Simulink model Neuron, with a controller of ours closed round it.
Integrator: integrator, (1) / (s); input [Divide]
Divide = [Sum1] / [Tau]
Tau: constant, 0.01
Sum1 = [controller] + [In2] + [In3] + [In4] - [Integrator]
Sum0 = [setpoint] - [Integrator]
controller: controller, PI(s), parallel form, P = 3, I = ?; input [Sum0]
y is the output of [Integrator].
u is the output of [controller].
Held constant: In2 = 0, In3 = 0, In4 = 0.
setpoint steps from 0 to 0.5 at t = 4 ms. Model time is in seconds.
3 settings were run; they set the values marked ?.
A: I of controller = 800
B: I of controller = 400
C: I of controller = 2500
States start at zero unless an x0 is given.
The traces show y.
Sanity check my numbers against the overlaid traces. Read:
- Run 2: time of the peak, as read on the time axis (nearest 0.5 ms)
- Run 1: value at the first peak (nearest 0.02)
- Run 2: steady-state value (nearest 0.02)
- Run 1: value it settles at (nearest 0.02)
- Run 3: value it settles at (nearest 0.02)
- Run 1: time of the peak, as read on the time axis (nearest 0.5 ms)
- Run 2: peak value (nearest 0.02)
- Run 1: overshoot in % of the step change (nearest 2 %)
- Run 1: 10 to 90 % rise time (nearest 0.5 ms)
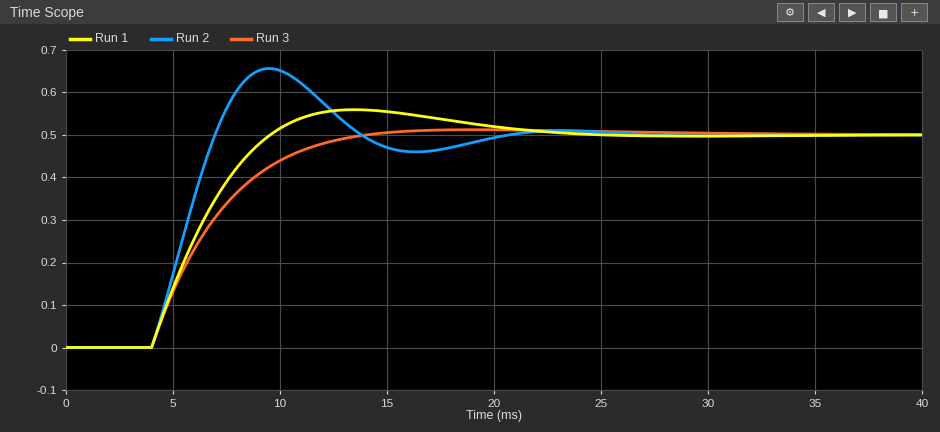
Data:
9.5 ms
0.56
0.50
0.50
0.50
13.5 ms
0.66
12 %
4.0 ms
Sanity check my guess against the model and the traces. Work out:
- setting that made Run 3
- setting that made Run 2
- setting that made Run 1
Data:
B
C
A
